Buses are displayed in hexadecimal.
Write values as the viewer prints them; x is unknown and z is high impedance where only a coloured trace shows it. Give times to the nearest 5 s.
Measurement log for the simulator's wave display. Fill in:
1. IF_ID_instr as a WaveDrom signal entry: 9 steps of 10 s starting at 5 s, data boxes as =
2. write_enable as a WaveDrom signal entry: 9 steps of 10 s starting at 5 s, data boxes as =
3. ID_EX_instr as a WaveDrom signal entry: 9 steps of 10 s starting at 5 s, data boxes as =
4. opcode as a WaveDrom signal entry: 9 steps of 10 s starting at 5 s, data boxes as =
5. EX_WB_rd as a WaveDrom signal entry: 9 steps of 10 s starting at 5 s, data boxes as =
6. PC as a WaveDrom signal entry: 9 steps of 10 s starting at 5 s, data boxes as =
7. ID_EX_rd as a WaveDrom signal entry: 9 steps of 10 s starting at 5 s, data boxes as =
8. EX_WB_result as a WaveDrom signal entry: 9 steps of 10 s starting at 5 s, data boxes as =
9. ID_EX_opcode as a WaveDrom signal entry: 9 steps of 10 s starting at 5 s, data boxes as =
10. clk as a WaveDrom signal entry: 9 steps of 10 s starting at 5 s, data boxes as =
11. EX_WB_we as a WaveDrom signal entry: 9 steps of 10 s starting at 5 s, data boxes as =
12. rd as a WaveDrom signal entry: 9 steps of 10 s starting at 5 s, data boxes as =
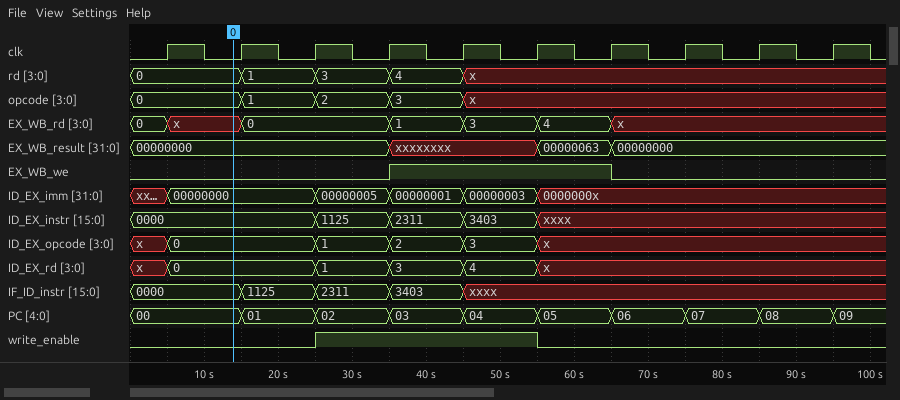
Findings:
{name: 'IF_ID_instr', wave: '====x....', data: '0000 1125 2311 3403'}
{name: 'write_enable', wave: '0.1..0...'}
{name: 'ID_EX_instr', wave: '=.===x...', data: '0000 1125 2311 3403'}
{name: 'opcode', wave: '====x....', data: '0 1 2 3'}
{name: 'EX_WB_rd', wave: 'x=.===x..', data: '0 1 3 4'}
{name: 'PC', wave: '=========', data: '00 01 02 03 04 05 06 07 08'}
{name: 'ID_EX_rd', wave: '=.===x...', data: '0 1 3 4'}
{name: 'EX_WB_result', wave: '=..x.==..', data: '00000000 00000063 00000000'}
{name: 'ID_EX_opcode', wave: '=.===x...', data: '0 1 2 3'}
{name: 'clk', wave: 'p........'}
{name: 'EX_WB_we', wave: '0..1..0..'}
{name: 'rd', wave: '====x....', data: '0 1 3 4'}
